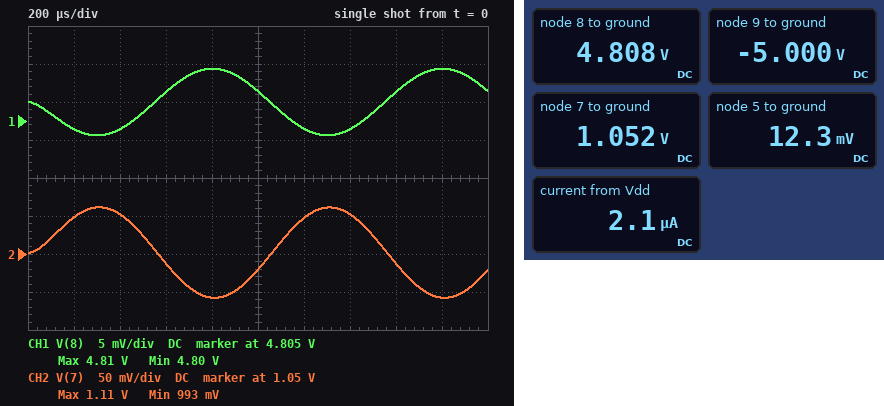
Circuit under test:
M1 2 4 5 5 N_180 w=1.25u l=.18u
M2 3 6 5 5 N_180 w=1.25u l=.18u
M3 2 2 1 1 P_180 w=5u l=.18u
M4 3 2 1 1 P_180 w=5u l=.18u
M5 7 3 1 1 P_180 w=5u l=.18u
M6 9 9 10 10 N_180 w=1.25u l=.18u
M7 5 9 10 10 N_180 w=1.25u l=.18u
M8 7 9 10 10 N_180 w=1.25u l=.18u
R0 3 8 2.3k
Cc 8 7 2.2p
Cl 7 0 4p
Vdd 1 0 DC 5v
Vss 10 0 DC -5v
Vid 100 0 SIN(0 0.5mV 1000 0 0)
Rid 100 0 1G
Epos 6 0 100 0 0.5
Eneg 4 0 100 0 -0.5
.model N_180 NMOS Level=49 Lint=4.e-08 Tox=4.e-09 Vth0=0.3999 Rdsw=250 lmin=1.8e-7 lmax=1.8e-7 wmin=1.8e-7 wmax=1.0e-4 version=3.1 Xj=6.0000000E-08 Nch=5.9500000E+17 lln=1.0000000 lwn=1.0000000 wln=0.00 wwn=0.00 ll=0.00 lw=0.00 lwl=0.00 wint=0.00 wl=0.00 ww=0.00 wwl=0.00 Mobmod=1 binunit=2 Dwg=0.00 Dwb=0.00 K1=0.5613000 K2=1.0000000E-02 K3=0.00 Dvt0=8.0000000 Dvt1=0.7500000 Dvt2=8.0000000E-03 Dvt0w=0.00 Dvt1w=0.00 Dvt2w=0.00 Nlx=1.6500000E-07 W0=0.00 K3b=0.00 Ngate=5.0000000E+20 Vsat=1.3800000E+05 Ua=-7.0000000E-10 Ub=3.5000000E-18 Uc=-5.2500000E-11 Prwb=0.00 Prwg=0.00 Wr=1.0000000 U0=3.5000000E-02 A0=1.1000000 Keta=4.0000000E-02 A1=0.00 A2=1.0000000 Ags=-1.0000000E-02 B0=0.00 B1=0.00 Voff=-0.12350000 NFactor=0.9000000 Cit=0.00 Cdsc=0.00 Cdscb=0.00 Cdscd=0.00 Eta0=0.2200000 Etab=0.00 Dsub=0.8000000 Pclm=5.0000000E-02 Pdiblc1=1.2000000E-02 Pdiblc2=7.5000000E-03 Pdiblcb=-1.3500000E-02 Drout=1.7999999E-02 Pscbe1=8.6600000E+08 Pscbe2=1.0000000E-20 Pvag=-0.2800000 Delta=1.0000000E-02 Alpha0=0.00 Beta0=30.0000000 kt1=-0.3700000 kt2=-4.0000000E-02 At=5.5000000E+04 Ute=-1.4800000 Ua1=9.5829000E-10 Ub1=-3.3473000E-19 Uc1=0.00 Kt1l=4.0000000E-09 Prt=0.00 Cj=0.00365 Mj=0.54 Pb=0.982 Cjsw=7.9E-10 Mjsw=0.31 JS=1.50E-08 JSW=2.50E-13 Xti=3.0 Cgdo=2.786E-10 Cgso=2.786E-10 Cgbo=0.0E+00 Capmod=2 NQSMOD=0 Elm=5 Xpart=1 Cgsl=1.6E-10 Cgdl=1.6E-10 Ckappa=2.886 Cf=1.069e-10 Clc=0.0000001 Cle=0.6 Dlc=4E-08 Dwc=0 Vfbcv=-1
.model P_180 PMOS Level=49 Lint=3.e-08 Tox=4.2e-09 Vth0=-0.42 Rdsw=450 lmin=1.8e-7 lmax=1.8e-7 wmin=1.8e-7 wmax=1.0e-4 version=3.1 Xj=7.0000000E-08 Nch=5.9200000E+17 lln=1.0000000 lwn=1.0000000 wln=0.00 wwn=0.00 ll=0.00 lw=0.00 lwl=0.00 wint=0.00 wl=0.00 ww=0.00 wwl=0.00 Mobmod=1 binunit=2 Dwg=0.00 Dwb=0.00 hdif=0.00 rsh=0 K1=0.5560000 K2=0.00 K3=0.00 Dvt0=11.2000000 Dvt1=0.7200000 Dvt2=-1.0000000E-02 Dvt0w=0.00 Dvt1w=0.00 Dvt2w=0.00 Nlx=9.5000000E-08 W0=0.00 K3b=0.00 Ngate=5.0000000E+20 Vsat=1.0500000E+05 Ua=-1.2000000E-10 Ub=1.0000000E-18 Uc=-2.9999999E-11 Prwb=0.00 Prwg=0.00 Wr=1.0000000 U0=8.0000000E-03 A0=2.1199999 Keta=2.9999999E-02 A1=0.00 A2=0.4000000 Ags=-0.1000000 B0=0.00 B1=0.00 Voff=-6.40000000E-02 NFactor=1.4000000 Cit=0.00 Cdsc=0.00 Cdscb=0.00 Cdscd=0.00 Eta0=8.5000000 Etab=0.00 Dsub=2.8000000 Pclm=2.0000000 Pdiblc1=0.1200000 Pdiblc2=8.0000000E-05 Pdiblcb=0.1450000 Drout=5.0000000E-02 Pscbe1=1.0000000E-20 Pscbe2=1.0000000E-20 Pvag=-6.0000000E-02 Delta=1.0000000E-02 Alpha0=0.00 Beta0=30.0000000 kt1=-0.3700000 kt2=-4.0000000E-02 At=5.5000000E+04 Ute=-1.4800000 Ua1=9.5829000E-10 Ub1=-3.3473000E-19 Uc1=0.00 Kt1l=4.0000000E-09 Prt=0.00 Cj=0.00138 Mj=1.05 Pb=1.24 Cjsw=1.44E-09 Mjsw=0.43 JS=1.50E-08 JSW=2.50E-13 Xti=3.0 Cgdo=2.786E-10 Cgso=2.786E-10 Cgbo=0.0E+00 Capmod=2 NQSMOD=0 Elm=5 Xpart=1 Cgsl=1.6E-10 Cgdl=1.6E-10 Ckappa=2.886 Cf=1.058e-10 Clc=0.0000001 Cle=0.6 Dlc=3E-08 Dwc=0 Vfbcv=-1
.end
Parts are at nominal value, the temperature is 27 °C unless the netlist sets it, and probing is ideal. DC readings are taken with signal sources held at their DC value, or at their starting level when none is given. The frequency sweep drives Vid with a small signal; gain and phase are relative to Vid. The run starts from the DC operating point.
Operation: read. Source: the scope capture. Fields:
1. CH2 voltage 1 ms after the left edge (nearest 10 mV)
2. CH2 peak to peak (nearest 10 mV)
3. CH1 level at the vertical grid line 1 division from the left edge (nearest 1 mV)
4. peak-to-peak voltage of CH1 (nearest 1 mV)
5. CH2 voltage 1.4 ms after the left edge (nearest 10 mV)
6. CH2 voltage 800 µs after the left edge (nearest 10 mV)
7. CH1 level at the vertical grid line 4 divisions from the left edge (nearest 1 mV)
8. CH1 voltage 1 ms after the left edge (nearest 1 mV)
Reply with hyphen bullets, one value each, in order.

- 1.03 V
- 120 mV
- 4.804 V
- 9 mV
- 1.10 V
- 990 mV
- 4.812 V
- 4.809 V
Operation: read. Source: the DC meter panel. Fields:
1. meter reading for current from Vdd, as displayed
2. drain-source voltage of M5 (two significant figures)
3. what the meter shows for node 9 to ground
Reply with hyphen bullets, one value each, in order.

- 2.1 µA
- -3.9 V
- -5.000 V
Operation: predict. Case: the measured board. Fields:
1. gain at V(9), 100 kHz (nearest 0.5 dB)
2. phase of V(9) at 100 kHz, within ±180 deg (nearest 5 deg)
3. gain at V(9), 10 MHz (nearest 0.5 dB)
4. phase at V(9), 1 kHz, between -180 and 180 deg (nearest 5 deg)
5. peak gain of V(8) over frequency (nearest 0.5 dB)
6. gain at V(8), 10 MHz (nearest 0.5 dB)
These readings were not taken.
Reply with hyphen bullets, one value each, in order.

- -10.0 dB
- -75 deg
- -55.0 dB
- 65 deg
- 19.5 dB
- -26.0 dB
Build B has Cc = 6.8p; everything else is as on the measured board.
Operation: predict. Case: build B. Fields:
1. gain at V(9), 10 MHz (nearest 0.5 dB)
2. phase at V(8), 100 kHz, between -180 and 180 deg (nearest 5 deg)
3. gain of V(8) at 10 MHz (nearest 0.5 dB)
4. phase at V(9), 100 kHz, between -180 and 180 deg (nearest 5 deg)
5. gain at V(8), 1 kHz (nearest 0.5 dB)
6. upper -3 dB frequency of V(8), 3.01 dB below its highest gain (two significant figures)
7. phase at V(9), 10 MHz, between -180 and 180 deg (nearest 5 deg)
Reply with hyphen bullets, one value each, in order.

- -54.0 dB
- 130 deg
- -31.5 dB
- -80 deg
- 15.5 dB
- 820 Hz
- 55 deg
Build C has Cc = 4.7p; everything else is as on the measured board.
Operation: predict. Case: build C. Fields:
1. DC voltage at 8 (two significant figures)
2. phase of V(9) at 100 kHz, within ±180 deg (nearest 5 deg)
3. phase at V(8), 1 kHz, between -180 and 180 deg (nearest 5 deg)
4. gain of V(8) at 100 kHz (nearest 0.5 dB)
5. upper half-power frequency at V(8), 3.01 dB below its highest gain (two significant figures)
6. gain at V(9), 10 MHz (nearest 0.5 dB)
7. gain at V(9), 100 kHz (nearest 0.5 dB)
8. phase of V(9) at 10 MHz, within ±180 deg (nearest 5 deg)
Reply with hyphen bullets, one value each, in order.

- 4.8 V
- -80 deg
- 145 deg
- -9.5 dB
- 1.2 kHz
- -54.5 dB
- -16.5 dB
- 55 deg
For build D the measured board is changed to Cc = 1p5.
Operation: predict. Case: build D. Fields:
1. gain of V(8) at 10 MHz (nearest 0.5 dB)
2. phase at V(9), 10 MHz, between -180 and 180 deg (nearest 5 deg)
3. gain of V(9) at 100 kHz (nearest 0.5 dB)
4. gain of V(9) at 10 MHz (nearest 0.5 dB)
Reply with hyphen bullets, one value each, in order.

- -24.0 dB
- 75 deg
- -6.5 dB
- -55.5 dB
